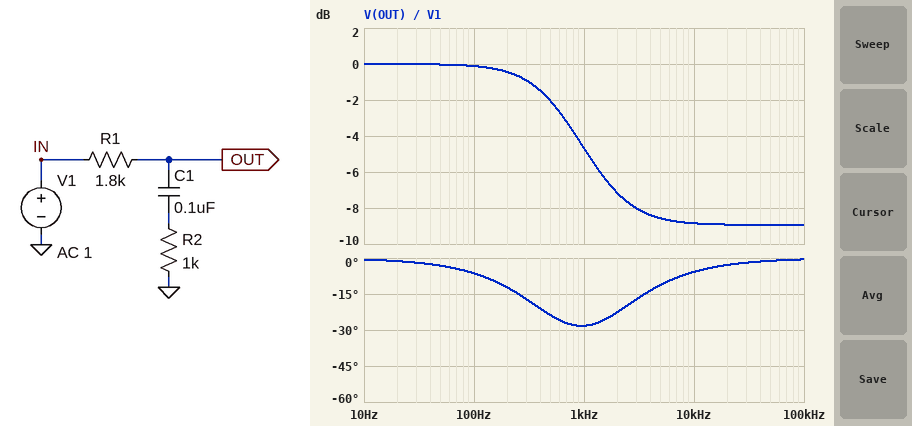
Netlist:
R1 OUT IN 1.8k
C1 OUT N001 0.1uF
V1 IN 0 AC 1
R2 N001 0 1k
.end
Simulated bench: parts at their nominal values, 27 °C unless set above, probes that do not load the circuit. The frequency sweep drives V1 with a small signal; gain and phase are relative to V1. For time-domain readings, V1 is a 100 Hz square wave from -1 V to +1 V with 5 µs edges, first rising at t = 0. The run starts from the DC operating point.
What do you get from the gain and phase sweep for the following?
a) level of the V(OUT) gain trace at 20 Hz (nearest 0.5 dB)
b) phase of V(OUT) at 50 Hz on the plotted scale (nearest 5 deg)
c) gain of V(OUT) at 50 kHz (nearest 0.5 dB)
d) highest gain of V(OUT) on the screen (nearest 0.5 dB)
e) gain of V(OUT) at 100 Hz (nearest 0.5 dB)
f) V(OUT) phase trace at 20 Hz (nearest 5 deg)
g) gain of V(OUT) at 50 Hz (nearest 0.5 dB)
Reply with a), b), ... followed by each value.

a) 0 dB
b) -5 deg
c) -9.0 dB
d) 0 dB
e) 0 dB
f) 0 deg
g) 0 dB
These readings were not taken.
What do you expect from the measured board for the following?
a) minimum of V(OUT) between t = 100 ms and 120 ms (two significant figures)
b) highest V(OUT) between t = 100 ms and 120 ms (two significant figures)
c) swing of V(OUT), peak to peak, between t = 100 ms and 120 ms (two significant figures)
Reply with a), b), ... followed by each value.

a) -1.0 V
b) 1.0 V
c) 2.0 V
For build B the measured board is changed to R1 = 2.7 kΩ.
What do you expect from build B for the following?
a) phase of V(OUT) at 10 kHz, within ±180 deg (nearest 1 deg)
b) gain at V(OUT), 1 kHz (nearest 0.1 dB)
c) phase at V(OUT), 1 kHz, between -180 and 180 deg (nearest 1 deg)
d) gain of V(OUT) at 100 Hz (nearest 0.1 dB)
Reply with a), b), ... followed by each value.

a) -7 deg
b) -6.6 dB
c) -35 deg
d) -0.2 dB
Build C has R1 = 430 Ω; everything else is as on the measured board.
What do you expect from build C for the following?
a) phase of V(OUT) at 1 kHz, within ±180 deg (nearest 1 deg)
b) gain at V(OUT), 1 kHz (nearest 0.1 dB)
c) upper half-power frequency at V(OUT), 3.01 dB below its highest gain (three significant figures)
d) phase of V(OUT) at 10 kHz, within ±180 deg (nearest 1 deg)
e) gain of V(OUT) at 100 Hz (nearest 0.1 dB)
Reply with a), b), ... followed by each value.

a) -10 deg
b) -1.1 dB
c) 7.51 kHz
d) -3 deg
e) 0 dB
